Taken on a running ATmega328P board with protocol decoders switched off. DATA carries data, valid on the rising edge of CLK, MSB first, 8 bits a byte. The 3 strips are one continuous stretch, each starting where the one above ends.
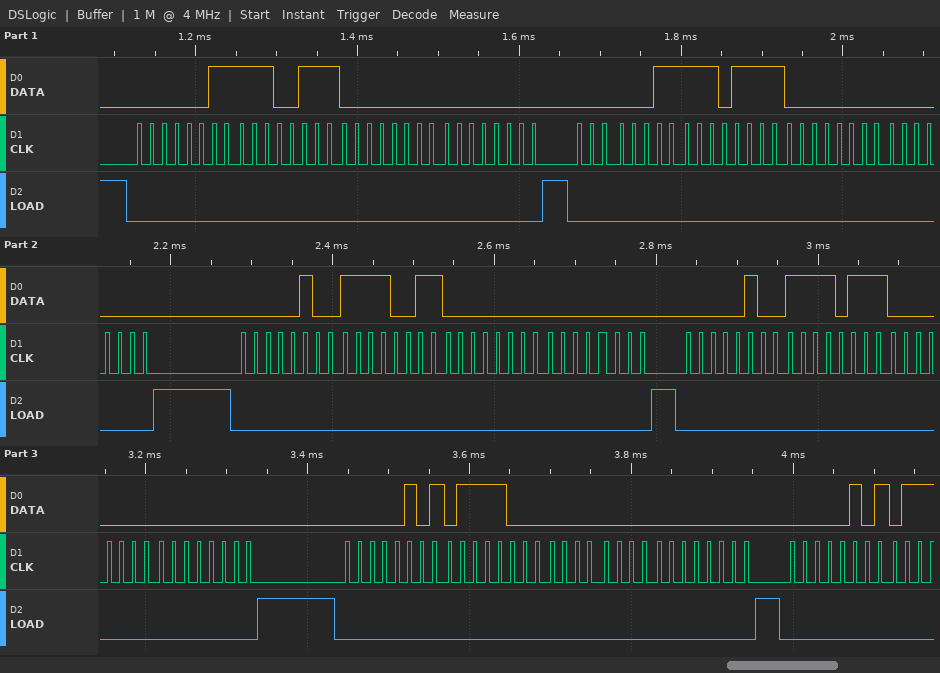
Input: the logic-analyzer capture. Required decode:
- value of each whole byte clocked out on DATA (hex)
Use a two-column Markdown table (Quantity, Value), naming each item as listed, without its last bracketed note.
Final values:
| Quantity | Value |
|---|---|
| value of each whole byte clocked out on DATA | 0x03 0xE7 0x00 0x00 0x03 0xEF 0x00 0x00 0x04 0xF3 0x00 0x00 0x04 0xF7 0x00 0x00 0x05 0x78 0x00 0x00 0x05 |
